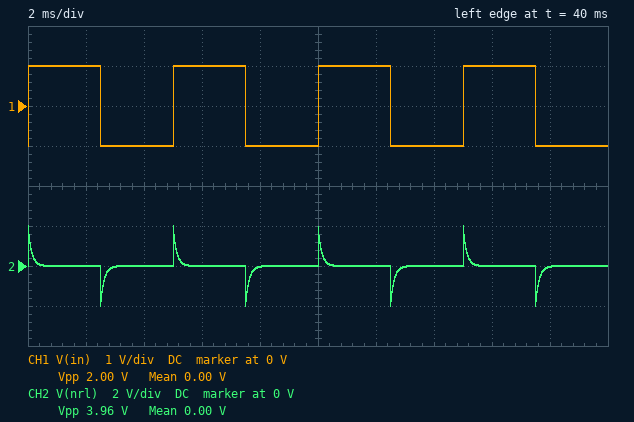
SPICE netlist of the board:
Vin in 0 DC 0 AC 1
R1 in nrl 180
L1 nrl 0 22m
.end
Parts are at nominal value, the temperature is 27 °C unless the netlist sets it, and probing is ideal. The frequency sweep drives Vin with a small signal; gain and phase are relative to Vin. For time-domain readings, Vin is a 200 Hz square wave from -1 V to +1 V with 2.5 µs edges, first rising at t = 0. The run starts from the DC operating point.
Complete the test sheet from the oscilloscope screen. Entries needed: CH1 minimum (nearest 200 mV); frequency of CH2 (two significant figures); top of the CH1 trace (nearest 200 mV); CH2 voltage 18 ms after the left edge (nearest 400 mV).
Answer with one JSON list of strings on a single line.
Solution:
["-1.0 V", "200 Hz", "1.0 V", "0 V"]
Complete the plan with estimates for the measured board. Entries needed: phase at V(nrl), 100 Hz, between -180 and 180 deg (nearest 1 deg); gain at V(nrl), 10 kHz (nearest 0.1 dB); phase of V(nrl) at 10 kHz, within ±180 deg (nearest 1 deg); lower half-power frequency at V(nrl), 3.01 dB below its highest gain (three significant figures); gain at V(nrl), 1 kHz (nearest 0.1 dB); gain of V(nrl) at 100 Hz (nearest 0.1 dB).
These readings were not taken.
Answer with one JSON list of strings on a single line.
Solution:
["86 deg", "-0.1 dB", "7 deg", "1.30 kHz", "-4.3 dB", "-22.3 dB"]
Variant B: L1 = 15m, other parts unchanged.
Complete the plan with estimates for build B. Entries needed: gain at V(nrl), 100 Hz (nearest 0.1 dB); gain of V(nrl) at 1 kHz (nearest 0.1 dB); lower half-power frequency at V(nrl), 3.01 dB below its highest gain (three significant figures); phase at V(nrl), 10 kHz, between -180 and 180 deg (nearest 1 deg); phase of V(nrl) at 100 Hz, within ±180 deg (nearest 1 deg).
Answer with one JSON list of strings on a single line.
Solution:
["-25.6 dB", "-6.7 dB", "1.91 kHz", "11 deg", "87 deg"]
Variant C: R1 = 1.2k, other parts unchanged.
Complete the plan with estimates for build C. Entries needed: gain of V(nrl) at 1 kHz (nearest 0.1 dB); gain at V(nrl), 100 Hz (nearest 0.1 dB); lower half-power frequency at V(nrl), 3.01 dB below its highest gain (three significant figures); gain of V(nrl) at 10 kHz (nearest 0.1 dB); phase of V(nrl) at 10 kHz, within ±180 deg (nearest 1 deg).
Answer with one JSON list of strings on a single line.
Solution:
["-18.8 dB", "-38.8 dB", "8.68 kHz", "-2.4 dB", "41 deg"]
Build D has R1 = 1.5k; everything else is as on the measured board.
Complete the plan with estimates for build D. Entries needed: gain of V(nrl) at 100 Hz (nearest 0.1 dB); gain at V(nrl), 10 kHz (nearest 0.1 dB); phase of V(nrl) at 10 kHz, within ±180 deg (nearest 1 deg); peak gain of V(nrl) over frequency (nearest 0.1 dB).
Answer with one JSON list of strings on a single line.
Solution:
["-40.7 dB", "-3.4 dB", "47 deg", "0 dB"]
